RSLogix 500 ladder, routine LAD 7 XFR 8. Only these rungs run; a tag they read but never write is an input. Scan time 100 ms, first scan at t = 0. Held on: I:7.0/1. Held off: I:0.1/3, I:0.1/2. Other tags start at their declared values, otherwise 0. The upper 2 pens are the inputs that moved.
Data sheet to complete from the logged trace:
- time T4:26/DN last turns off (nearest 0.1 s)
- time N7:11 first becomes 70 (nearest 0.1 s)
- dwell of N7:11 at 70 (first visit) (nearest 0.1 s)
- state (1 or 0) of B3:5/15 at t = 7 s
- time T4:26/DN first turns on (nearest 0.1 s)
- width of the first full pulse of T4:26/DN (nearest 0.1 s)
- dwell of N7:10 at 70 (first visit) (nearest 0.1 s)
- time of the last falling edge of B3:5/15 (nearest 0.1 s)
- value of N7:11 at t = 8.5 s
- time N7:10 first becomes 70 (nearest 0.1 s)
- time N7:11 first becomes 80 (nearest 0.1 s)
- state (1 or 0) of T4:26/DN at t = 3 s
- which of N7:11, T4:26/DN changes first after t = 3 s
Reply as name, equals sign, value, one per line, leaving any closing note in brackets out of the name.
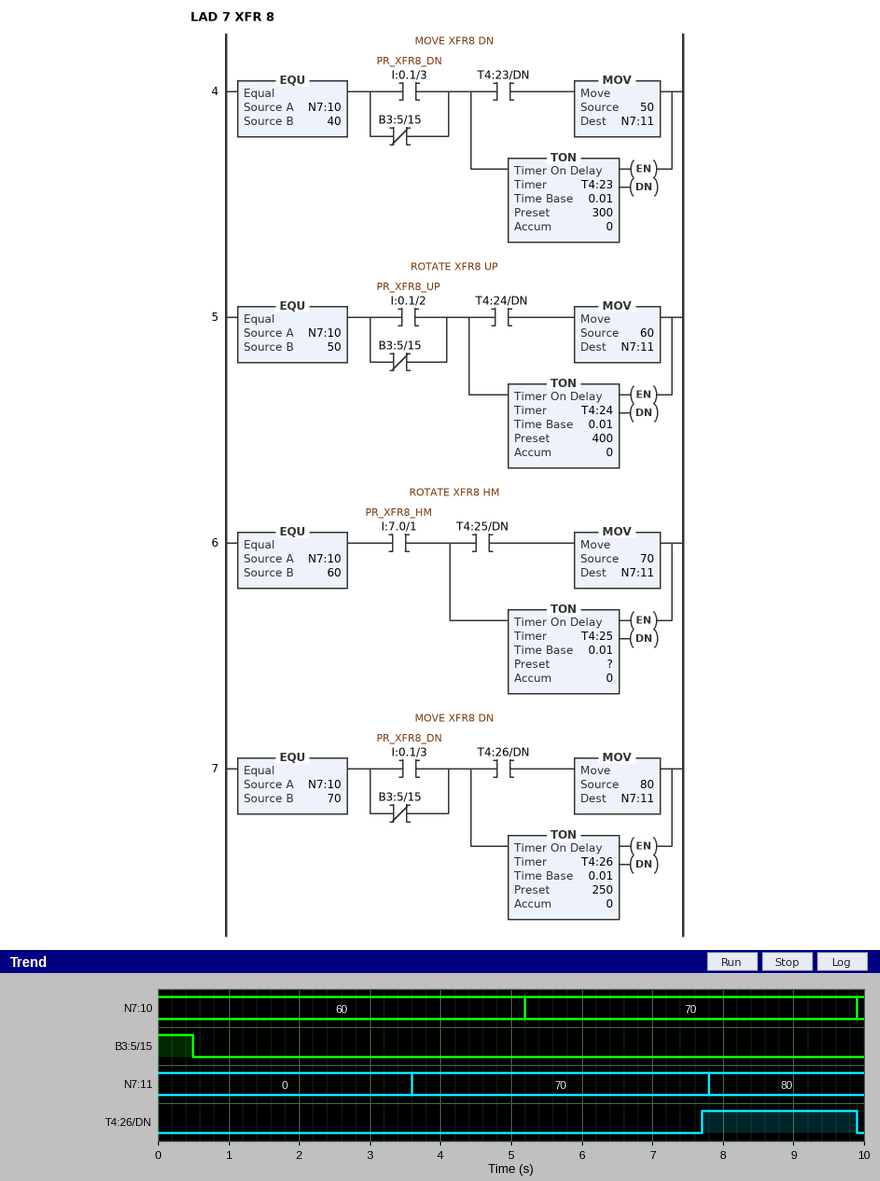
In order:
time T4:26/DN last turns off = 9.9 s
time N7:11 first becomes 70 = 3.6 s
dwell of N7:11 at 70 (first visit) = 4.2 s
state (1 or 0) of B3:5/15 at t = 7 s = 0
time T4:26/DN first turns on = 7.7 s
width of the first full pulse of T4:26/DN = 2.2 s
dwell of N7:10 at 70 (first visit) = 4.7 s
time of the last falling edge of B3:5/15 = 0.5 s
value of N7:11 at t = 8.5 s = 80
time N7:10 first becomes 70 = 5.2 s
time N7:11 first becomes 80 = 7.8 s
state (1 or 0) of T4:26/DN at t = 3 s = 0
which of N7:11, T4:26/DN changes first after t = 3 s = N7:11
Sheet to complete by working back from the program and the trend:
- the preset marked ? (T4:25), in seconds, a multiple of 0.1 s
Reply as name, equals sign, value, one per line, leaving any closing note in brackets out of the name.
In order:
the preset marked ? (T4:25), in seconds, a multiple of 0.1 s = 3.5 s
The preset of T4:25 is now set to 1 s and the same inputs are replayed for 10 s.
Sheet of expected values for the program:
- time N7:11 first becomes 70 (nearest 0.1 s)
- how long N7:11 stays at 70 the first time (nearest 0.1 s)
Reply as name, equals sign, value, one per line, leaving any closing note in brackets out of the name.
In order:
time N7:11 first becomes 70 = 1.1 s
how long N7:11 stays at 70 the first time = 6.7 s
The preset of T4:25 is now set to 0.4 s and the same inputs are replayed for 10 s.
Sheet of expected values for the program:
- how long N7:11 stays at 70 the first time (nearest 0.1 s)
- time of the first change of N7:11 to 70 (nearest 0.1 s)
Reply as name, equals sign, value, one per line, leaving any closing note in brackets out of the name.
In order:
how long N7:11 stays at 70 the first time = 7.3 s
time of the first change of N7:11 to 70 = 0.5 s
